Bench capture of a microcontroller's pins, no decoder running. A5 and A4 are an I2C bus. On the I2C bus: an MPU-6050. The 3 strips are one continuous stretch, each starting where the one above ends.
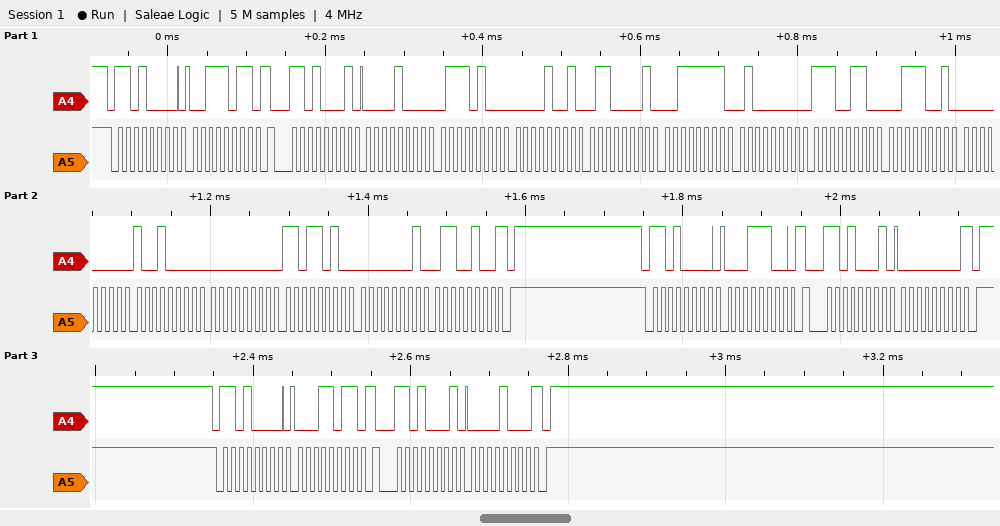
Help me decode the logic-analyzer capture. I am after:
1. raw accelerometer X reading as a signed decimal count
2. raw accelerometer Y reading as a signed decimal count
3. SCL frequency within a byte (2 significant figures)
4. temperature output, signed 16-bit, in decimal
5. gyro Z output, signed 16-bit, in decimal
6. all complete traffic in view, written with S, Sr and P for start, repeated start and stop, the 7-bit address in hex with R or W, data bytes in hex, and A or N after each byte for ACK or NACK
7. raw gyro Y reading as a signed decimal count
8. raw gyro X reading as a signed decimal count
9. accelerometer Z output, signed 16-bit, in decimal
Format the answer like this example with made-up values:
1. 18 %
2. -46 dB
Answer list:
1. 2164
2. 2401
3. 100 kHz
4. -6599
5. 356
6. S 68W A 3B A Sr 68R A 08 A 74 A 09 A 61 A 3F A 40 A E6 A 39 A 00 A 90 A 00 A DA A 01 A 64 N P S 68W A 1C A Sr 68R A 00 N P S 68W A 1B A Sr 68R A 08 N P
7. 218
8. 144
9. 16192
